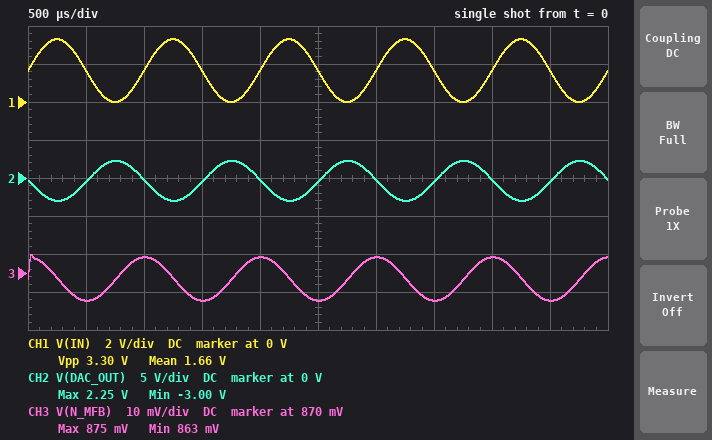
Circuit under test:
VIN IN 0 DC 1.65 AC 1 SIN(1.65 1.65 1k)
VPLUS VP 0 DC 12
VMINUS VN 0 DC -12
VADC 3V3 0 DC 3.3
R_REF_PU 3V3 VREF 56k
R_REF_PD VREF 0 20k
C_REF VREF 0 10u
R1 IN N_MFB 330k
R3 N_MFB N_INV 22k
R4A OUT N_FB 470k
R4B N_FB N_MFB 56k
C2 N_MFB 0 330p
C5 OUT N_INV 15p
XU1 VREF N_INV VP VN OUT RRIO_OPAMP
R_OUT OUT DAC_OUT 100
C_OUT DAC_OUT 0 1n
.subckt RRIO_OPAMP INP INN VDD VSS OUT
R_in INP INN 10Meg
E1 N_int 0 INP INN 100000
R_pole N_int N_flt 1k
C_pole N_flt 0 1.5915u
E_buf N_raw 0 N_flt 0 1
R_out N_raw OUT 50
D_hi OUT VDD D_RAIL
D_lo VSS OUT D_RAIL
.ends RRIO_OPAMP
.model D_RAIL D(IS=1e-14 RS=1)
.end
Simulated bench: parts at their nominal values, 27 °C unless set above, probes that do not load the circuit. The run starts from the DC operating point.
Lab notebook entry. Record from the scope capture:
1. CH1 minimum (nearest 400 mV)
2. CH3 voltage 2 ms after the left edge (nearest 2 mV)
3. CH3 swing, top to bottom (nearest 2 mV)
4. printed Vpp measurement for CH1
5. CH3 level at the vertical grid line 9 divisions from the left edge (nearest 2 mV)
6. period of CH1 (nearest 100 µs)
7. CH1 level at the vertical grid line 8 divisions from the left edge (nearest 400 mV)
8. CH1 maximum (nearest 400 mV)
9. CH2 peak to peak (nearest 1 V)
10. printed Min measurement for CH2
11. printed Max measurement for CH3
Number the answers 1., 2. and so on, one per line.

1. 0 V
2. 874 mV
3. 12 mV
4. 3.30 V
5. 862 mV
6. 1.0 ms
7. 1.6 V
8. 3.2 V
9. 5 V
10. -3.00 V
11. 875 mV
